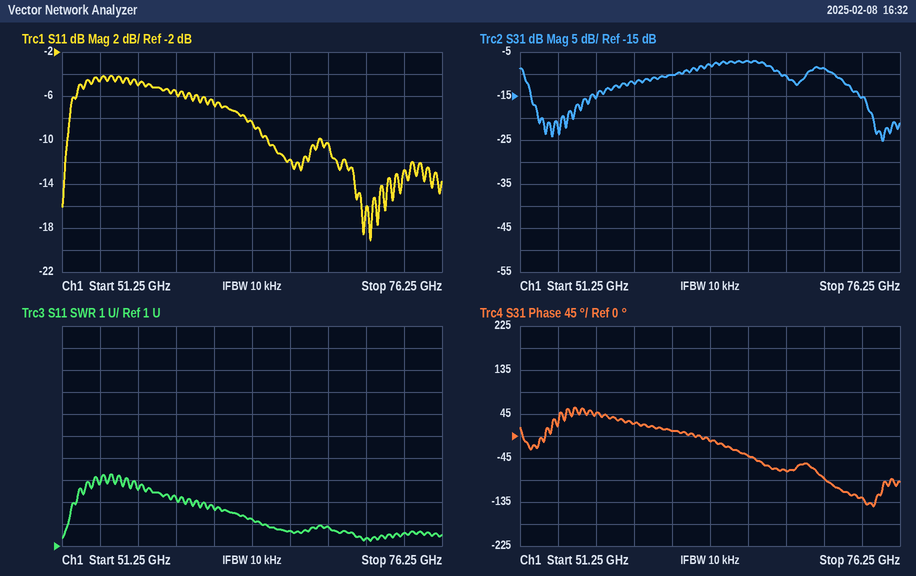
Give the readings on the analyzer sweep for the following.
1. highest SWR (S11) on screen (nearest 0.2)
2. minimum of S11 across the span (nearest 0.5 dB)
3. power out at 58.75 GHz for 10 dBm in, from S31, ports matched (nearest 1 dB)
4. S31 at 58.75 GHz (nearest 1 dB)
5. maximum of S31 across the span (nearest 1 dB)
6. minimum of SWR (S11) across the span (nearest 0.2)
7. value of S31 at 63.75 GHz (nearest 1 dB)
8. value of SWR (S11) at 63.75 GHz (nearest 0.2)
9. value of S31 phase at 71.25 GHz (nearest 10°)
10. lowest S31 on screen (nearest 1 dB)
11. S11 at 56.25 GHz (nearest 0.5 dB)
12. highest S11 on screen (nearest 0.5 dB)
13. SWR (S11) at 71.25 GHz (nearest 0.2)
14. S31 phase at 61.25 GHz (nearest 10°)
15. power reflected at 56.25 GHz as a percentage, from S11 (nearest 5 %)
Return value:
4.2
-19.0 dB
-2 dBm
-12 dB
-7 dB
1.2
-8 dB
2.2
-90°
-25 dB
-5.0 dB
-4.0 dB
1.4
10°
30 %
